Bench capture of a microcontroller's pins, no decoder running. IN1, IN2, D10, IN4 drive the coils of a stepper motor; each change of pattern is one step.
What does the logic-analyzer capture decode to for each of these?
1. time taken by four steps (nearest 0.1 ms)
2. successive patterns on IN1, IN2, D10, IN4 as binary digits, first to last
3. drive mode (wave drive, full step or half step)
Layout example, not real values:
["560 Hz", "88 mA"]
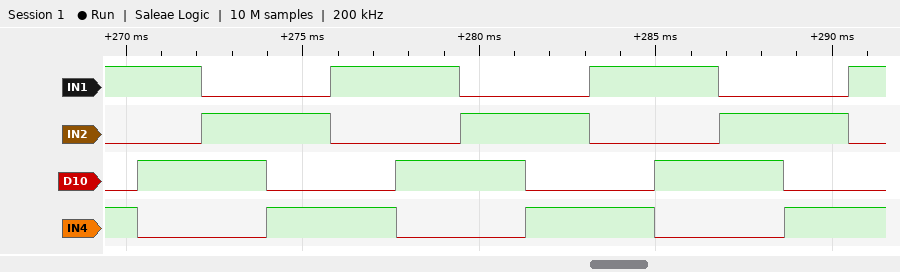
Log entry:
["7.3 ms", "1001 1010 0110 0101 1001 1010 0110 0101 1001 1010 0110 0101 1001", "full step"]
